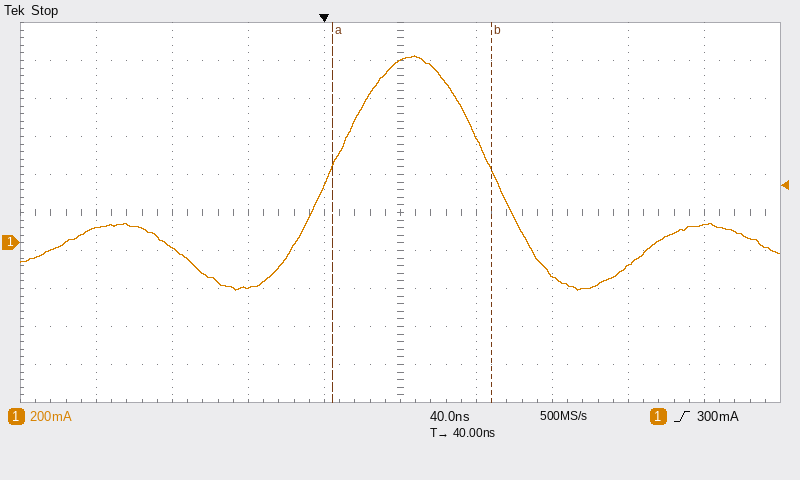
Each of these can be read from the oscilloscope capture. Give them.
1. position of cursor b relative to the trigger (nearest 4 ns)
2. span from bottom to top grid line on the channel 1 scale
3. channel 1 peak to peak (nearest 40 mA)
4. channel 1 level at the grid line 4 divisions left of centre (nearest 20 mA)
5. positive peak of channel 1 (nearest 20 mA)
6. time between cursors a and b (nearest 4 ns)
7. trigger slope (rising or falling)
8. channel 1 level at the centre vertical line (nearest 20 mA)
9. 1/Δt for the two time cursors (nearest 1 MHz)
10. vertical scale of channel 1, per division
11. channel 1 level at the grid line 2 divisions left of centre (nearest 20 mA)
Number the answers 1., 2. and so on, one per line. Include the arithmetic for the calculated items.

1. +88 ns
2. 2 A
3. 1.24 A
4. 80 mA
5. 980 mA
6. 84 ns
7. rising
8. 960 mA
9. 1 / 84 ns ≈ 12 MHz
10. 200 mA
11. -240 mA
